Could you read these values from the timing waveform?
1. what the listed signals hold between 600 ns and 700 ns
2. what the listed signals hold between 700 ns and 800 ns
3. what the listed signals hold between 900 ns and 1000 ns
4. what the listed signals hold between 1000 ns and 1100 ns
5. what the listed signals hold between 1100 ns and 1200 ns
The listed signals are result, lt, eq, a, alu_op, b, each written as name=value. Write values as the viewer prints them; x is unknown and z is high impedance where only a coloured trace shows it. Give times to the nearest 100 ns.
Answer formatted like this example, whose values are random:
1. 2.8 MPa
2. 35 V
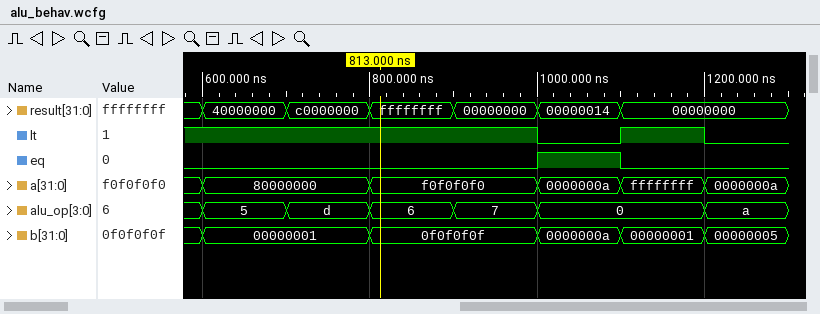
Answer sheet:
1. result=40000000, lt=1, eq=0, a=80000000, alu_op=5, b=00000001
2. result=c0000000, lt=1, eq=0, a=80000000, alu_op=d, b=00000001
3. result=00000000, lt=1, eq=0, a=f0f0f0f0, alu_op=7, b=0f0f0f0f
4. result=00000014, lt=0, eq=1, a=0000000a, alu_op=0, b=0000000a
5. result=00000000, lt=1, eq=0, a=ffffffff, alu_op=0, b=00000001
